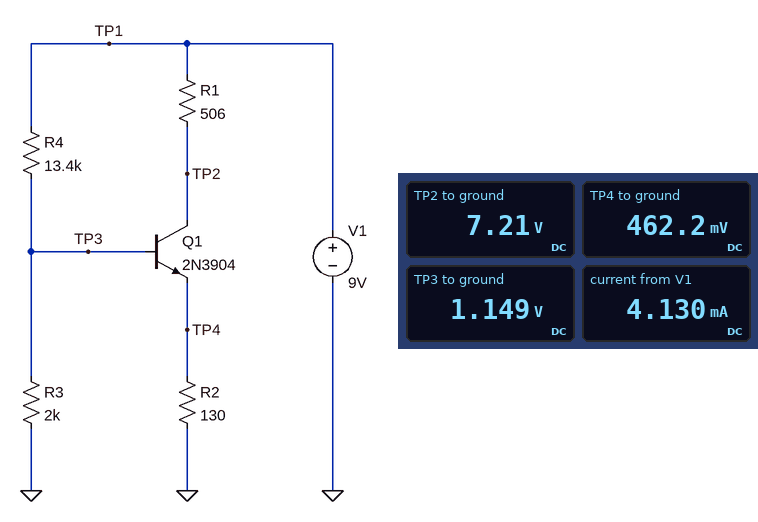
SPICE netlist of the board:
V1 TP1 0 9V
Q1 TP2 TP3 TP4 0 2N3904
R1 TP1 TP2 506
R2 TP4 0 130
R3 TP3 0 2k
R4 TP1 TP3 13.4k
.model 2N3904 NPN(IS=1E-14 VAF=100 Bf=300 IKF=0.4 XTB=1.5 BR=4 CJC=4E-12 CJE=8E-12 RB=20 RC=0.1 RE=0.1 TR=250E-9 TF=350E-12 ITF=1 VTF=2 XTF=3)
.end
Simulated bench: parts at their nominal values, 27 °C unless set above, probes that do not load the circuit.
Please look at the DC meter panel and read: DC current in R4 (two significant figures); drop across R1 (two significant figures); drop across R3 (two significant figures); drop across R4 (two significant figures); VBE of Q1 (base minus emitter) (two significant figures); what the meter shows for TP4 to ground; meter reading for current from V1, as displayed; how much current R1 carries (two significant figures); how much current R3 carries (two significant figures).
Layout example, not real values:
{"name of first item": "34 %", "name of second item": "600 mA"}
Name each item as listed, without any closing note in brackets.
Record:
{"DC current in R4": "590 µA", "drop across R1": "1.8 V", "drop across R3": "1.1 V", "drop across R4": "7.9 V", "VBE of Q1 (base minus emitter)": "690 mV", "what the meter shows for TP4 to ground": "462.2 mV", "meter reading for current from V1, as displayed": "4.130 mA", "how much current R1 carries": "3.5 mA", "how much current R3 carries": "570 µA"}
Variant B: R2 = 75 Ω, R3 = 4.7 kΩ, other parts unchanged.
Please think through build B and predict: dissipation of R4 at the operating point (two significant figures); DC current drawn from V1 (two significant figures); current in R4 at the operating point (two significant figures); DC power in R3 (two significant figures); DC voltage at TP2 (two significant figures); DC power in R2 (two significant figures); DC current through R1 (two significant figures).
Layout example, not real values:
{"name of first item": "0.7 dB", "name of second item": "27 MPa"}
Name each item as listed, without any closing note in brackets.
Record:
{"dissipation of R4 at the operating point": "3.8 mW", "DC current drawn from V1": "16 mA", "current in R4 at the operating point": "530 µA", "DC power in R3": "760 µW", "DC voltage at TP2": "1.3 V", "DC power in R2": "18 mW", "DC current through R1": "15 mA"}
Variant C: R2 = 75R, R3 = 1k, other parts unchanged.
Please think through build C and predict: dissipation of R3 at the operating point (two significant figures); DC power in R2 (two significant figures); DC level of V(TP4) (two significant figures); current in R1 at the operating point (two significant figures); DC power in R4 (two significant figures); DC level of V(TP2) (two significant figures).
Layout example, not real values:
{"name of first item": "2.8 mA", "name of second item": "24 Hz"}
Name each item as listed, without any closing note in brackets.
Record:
{"dissipation of R3 at the operating point": "390 µW", "DC power in R2": "2.7 µW", "DC level of V(TP4)": "14 mV", "current in R1 at the operating point": "190 µA", "DC power in R4": "5.2 mW", "DC level of V(TP2)": "8.9 V"}
